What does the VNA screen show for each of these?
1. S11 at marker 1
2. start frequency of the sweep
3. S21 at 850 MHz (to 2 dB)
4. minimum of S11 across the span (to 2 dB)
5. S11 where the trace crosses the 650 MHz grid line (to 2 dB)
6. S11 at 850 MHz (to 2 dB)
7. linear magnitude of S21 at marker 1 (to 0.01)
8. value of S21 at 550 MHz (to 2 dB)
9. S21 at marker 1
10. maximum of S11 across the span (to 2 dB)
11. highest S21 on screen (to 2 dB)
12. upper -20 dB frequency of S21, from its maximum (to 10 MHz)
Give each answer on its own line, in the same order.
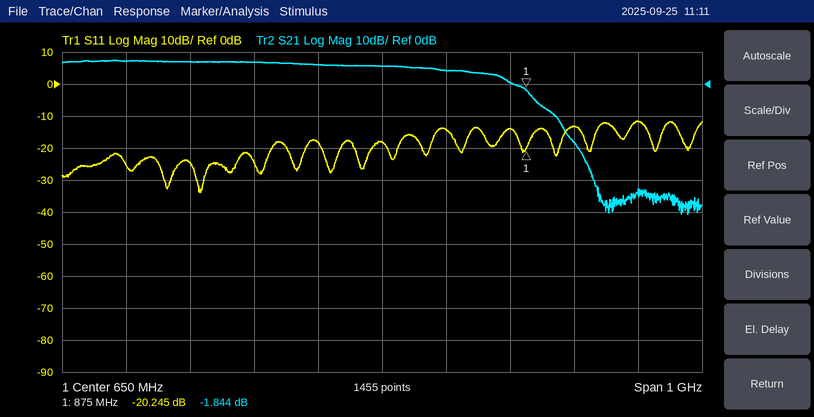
-20.245 dB
150 MHz
0 dB
-34 dB
-18 dB
-14 dB
0.81
6 dB
-1.844 dB
-12 dB
8 dB
930 MHz
